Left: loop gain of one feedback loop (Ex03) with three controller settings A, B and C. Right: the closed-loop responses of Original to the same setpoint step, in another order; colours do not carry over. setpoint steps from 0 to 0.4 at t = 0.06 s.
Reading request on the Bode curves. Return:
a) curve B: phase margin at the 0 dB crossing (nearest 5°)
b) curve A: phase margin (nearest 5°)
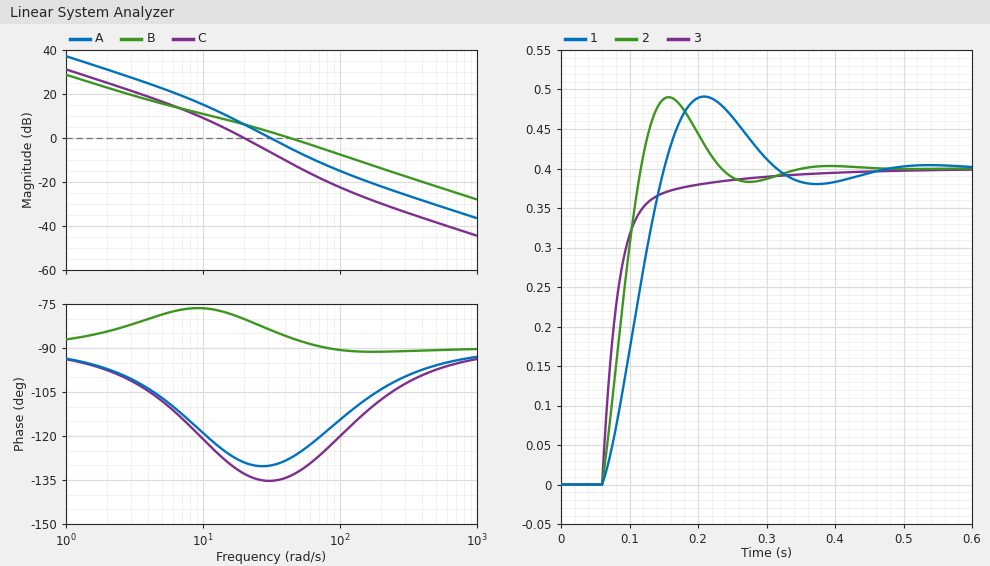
95°
50°
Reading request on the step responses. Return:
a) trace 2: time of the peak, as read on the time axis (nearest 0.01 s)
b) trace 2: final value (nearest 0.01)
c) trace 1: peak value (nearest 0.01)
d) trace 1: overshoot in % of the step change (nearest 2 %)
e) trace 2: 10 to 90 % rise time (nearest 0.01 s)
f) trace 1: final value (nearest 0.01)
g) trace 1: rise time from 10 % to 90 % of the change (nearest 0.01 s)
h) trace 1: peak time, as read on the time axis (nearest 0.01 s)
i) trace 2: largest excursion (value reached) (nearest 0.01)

0.16 s
0.40
0.49
22 %
0.04 s
0.40
0.07 s
0.21 s
0.49
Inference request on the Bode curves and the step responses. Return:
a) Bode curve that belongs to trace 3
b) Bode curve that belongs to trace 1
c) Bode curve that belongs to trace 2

B
C
A
